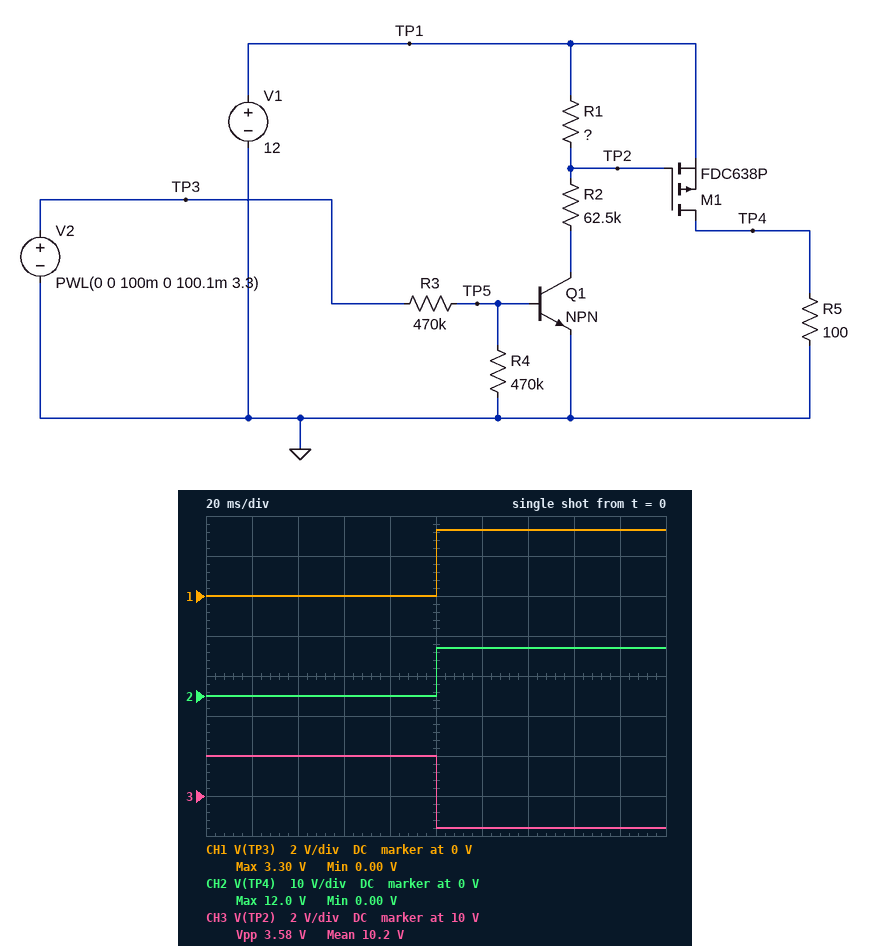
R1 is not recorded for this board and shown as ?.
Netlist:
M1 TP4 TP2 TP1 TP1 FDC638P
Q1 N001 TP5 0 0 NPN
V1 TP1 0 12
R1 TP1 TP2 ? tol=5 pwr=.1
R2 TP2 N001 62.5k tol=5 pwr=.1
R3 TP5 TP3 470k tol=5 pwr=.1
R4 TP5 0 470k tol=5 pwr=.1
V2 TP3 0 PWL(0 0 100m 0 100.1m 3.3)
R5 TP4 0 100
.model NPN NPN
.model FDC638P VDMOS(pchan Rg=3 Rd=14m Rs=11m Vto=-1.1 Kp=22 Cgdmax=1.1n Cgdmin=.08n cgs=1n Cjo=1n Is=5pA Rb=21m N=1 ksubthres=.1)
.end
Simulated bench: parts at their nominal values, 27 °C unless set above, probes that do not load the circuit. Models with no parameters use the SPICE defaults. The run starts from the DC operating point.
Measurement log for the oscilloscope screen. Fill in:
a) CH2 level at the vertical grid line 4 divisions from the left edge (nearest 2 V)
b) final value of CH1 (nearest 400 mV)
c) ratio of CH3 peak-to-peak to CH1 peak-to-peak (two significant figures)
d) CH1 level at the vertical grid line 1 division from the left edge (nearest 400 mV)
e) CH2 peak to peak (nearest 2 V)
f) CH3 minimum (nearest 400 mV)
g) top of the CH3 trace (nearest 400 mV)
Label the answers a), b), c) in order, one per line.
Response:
a) 0 V
b) 3.2 V
c) 1.1
d) 0 V
e) 12 V
f) 8.4 V
g) 12.0 V
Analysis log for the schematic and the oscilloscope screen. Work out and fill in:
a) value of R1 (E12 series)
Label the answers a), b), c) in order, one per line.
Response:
a) 27 kΩ
